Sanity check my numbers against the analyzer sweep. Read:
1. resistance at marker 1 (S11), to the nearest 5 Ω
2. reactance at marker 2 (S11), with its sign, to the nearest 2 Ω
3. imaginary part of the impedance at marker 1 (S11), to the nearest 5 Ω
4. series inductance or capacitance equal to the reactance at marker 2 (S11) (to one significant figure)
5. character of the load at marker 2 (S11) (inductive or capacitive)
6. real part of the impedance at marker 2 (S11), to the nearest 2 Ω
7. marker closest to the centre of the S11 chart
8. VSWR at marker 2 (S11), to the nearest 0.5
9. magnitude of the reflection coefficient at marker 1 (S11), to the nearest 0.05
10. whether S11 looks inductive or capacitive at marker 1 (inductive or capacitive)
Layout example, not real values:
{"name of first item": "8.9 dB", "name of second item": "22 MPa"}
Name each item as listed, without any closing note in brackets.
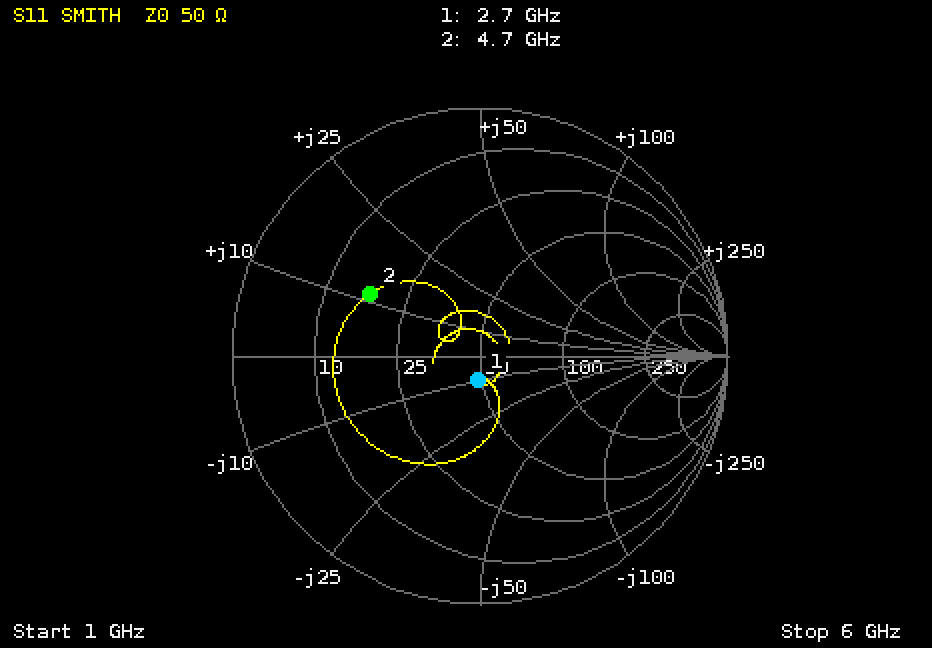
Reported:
{"resistance at marker 1 (S11), to the nearest 5 Ω": "50 Ω", "reactance at marker 2 (S11), with its sign, to the nearest 2 Ω": "+12 Ω", "imaginary part of the impedance at marker 1 (S11), to the nearest 5 Ω": "-10 Ω", "series inductance or capacitance equal to the reactance at marker 2 (S11)": "400 pH", "character of the load at marker 2 (S11)": "inductive", "real part of the impedance at marker 2 (S11), to the nearest 2 Ω": "18 Ω", "marker closest to the centre of the S11 chart": "marker 1", "VSWR at marker 2 (S11), to the nearest 0.5": "3.0", "magnitude of the reflection coefficient at marker 1 (S11), to the nearest 0.05": "0.10", "whether S11 looks inductive or capacitive at marker 1": "capacitive"}
